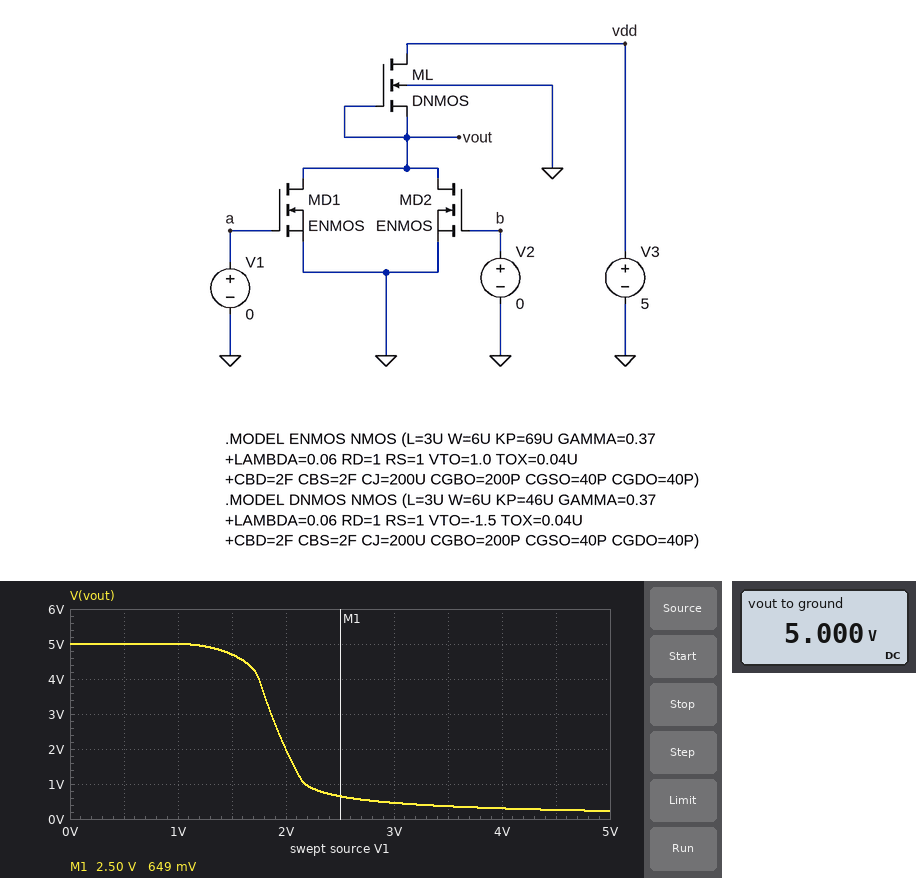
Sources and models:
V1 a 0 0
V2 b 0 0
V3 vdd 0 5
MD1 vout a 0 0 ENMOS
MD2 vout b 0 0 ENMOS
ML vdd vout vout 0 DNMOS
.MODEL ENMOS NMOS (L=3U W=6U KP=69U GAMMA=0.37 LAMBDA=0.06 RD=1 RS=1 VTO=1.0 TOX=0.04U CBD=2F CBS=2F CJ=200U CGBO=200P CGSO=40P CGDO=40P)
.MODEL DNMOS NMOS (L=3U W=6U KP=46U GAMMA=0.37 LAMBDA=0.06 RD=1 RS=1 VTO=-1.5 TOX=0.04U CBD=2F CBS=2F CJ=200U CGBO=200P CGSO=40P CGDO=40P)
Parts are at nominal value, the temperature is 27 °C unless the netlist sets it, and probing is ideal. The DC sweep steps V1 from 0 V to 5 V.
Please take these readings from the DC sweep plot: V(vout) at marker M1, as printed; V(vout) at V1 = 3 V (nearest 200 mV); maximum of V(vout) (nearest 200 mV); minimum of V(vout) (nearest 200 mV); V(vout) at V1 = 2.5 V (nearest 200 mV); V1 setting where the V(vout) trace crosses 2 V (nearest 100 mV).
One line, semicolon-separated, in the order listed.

649 mV; 400 mV; 5.0 V; 200 mV; 600 mV; 2.0 V
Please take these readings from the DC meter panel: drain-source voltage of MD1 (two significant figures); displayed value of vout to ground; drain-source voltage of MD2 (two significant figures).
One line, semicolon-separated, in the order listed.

5.0 V; 5.000 V; 5.0 V
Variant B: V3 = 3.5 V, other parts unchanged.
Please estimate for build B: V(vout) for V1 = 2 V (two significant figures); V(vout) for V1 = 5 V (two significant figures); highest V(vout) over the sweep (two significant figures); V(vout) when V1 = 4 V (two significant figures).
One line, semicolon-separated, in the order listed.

1.7 V; 210 mV; 3.5 V; 280 mV
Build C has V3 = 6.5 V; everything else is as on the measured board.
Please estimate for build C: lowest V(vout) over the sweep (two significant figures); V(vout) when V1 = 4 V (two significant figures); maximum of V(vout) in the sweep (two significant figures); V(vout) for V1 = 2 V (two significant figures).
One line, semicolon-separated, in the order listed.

240 mV; 320 mV; 6.5 V; 2.2 V
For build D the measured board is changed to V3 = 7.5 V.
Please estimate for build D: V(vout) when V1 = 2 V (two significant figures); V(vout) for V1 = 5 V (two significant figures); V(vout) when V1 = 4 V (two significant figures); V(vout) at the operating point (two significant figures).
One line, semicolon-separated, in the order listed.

2.4 V; 250 mV; 340 mV; 7.5 V
